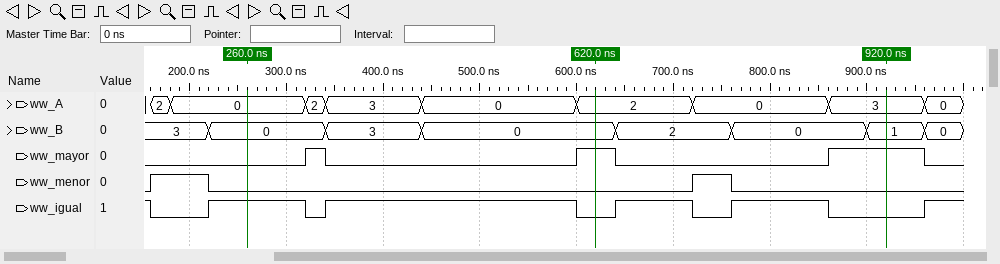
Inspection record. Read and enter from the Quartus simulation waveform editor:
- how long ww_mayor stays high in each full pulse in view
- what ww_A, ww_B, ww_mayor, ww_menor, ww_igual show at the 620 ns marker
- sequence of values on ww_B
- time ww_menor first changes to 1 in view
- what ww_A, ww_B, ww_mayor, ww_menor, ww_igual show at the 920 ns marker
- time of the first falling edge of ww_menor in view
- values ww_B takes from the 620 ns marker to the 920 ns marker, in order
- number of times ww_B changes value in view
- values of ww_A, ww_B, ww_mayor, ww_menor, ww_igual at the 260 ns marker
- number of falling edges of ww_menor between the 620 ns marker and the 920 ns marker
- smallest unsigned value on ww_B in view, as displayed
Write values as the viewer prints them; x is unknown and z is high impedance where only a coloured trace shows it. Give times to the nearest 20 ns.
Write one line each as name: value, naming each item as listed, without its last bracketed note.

how long ww_mayor stays high in each full pulse in view: 20 ns, 40 ns, 100 ns
what ww_A, ww_B, ww_mayor, ww_menor, ww_igual show at the 620 ns marker: ww_A=2, ww_B=0, ww_mayor=1, ww_menor=0, ww_igual=0
sequence of values on ww_B: 3, 0, 3, 0, 2, 0, 1, 0
time ww_menor first changes to 1 in view: 160 ns
what ww_A, ww_B, ww_mayor, ww_menor, ww_igual show at the 920 ns marker: ww_A=3, ww_B=1, ww_mayor=1, ww_menor=0, ww_igual=0
time of the first falling edge of ww_menor in view: 220 ns
values ww_B takes from the 620 ns marker to the 920 ns marker, in order: 0, 2, 0, 1
number of times ww_B changes value in view: 7
values of ww_A, ww_B, ww_mayor, ww_menor, ww_igual at the 260 ns marker: ww_A=0, ww_B=0, ww_mayor=0, ww_menor=0, ww_igual=1
number of falling edges of ww_menor between the 620 ns marker and the 920 ns marker: 1
smallest unsigned value on ww_B in view, as displayed: 0
